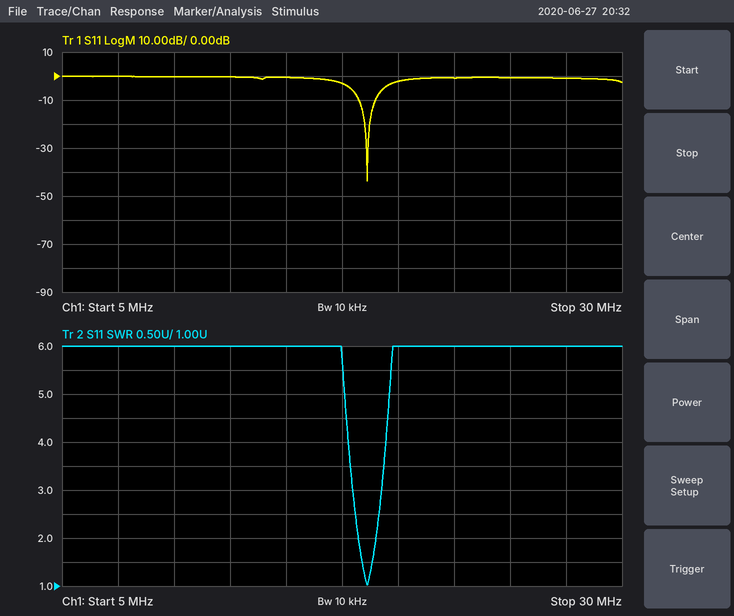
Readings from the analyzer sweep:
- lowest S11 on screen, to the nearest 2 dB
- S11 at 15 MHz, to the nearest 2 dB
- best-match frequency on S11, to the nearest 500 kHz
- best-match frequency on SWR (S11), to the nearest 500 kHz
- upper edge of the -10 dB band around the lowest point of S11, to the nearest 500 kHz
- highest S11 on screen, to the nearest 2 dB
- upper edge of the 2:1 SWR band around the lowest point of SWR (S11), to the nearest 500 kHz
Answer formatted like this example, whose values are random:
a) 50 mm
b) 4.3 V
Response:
a) -44 dB
b) 0 dB
c) 18.5 MHz
d) 18.5 MHz
e) 19.0 MHz
f) 0 dB
g) 19.0 MHz
